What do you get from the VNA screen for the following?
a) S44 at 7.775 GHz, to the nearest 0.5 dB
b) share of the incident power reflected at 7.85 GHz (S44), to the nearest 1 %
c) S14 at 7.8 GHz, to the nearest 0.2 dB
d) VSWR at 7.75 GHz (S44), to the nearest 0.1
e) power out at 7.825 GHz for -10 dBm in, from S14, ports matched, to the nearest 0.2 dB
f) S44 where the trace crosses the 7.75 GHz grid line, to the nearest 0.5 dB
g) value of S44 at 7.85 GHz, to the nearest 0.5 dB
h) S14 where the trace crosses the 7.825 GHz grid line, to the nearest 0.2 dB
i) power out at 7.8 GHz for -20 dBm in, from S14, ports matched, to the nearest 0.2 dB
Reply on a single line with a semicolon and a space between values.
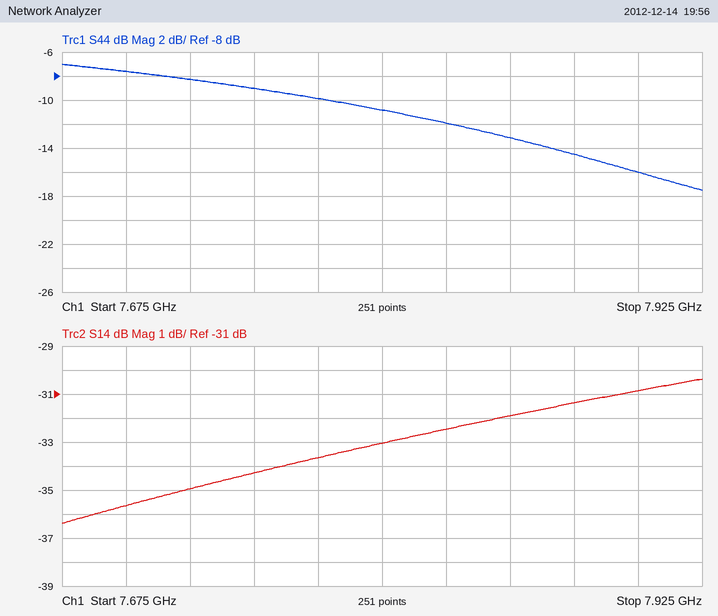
-10.0 dB; 5 %; -33.0 dB; 2.1; -42.4 dBm; -9.0 dB; -13.0 dB; -32.4 dB; -53.0 dBm
